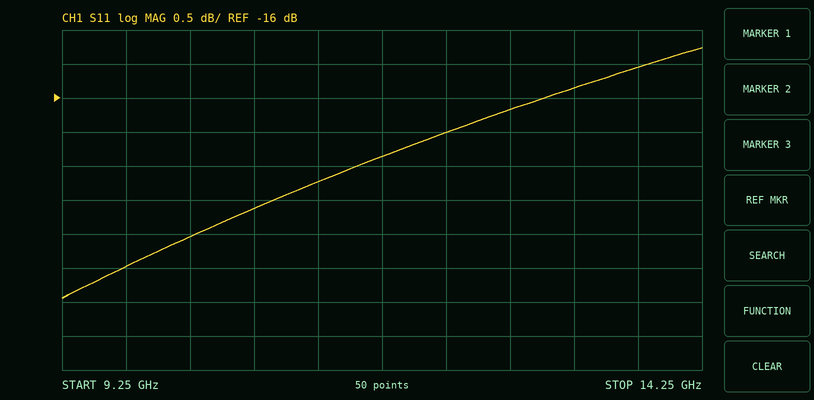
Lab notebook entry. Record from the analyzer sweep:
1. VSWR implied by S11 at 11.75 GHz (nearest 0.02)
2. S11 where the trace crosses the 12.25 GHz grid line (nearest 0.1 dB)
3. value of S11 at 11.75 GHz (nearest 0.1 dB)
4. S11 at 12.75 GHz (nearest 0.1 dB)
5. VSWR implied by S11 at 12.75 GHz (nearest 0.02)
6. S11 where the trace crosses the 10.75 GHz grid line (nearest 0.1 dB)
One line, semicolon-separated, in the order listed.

1.34; -16.5 dB; -16.9 dB; -16.2 dB; 1.36; -17.6 dB
